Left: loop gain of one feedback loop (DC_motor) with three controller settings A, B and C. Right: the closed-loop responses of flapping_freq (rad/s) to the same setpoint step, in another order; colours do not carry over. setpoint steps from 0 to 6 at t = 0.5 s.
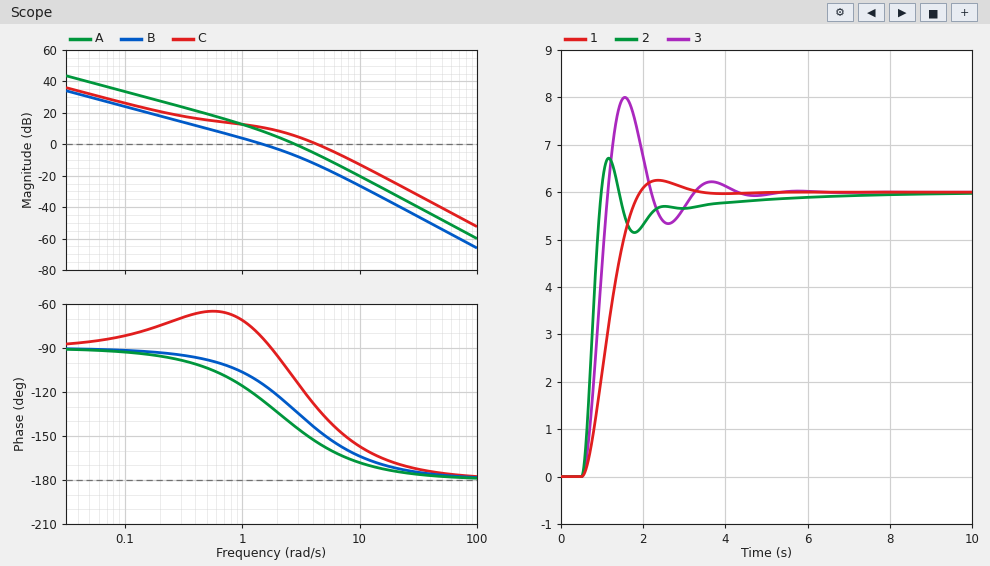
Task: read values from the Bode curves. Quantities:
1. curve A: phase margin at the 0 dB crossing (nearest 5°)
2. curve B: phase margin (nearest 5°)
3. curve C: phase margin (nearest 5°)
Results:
35°
65°
50°
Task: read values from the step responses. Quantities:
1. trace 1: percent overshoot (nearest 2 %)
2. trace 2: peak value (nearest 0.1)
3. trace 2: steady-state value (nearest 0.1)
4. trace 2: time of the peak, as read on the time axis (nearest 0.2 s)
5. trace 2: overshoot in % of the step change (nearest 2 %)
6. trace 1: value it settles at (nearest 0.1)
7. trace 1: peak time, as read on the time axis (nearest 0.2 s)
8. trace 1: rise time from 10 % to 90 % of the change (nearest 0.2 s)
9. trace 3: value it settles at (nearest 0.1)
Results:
4 %
6.7
6.0
1.2 s
12 %
6.0
2.4 s
1.0 s
6.0
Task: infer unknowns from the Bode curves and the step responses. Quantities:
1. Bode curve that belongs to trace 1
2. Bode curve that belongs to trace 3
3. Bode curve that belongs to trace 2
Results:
B
A
C
